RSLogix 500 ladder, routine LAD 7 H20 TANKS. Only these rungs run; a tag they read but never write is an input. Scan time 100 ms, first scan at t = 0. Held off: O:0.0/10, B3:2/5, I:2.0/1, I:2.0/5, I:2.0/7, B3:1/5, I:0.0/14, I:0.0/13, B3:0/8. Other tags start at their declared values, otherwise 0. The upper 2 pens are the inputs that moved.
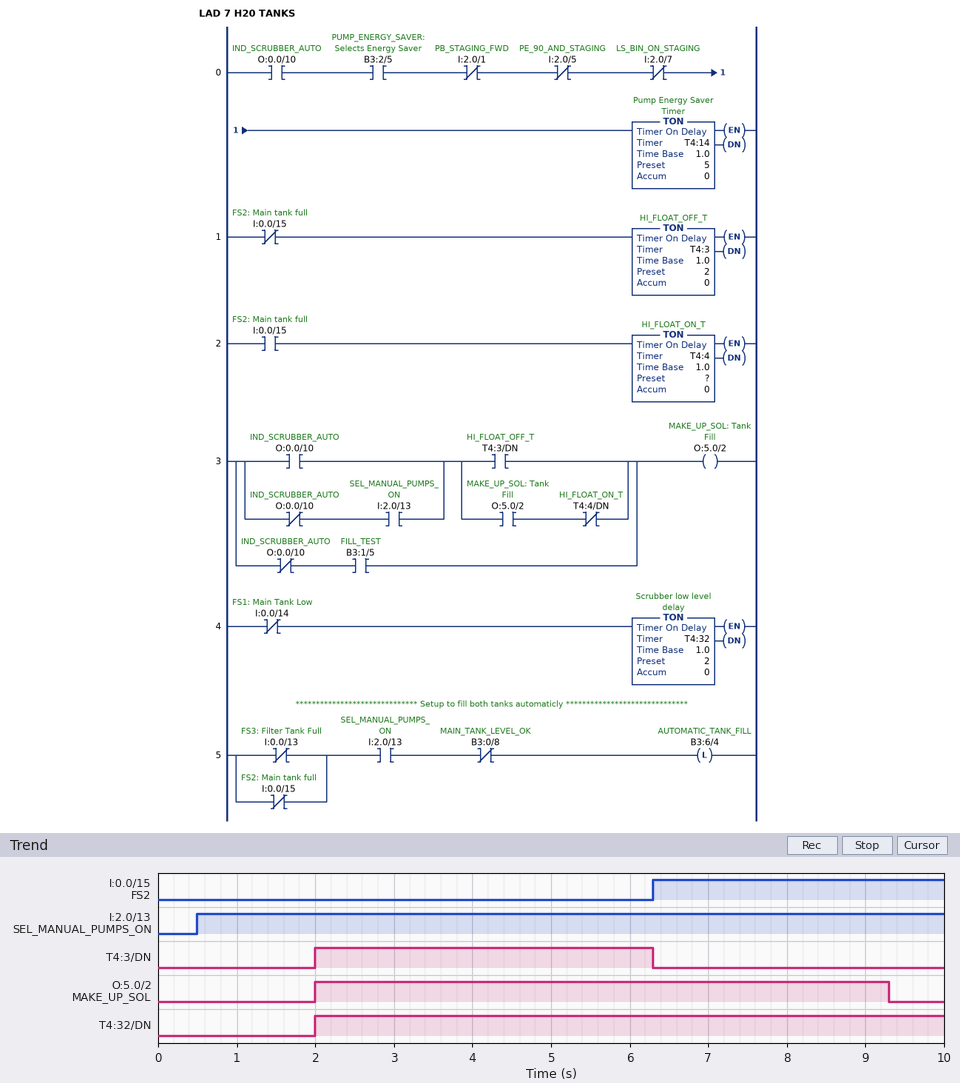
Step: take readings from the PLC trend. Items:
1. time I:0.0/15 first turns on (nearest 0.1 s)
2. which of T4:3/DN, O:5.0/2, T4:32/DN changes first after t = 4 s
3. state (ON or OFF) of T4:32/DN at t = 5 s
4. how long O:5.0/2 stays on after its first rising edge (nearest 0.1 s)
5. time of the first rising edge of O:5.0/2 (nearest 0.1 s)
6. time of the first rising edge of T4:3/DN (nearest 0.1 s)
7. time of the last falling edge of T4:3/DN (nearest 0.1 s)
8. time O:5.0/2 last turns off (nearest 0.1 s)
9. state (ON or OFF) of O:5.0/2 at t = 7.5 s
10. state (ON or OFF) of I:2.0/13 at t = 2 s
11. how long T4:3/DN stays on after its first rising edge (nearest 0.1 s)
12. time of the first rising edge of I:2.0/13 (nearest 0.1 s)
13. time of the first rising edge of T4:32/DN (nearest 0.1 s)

6.3 s
T4:3/DN
ON
7.3 s
2.0 s
2.0 s
6.3 s
9.3 s
ON
ON
4.3 s
0.5 s
2.0 s
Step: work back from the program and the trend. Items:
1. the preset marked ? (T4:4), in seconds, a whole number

3 s
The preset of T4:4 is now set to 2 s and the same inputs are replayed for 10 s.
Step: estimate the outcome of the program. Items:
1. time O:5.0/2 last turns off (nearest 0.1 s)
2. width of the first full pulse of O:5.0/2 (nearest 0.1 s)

8.3 s
6.3 s
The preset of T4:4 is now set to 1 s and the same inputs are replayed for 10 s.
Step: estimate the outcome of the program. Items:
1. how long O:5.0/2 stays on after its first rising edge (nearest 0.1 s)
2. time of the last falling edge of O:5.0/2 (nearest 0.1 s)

5.3 s
7.3 s
